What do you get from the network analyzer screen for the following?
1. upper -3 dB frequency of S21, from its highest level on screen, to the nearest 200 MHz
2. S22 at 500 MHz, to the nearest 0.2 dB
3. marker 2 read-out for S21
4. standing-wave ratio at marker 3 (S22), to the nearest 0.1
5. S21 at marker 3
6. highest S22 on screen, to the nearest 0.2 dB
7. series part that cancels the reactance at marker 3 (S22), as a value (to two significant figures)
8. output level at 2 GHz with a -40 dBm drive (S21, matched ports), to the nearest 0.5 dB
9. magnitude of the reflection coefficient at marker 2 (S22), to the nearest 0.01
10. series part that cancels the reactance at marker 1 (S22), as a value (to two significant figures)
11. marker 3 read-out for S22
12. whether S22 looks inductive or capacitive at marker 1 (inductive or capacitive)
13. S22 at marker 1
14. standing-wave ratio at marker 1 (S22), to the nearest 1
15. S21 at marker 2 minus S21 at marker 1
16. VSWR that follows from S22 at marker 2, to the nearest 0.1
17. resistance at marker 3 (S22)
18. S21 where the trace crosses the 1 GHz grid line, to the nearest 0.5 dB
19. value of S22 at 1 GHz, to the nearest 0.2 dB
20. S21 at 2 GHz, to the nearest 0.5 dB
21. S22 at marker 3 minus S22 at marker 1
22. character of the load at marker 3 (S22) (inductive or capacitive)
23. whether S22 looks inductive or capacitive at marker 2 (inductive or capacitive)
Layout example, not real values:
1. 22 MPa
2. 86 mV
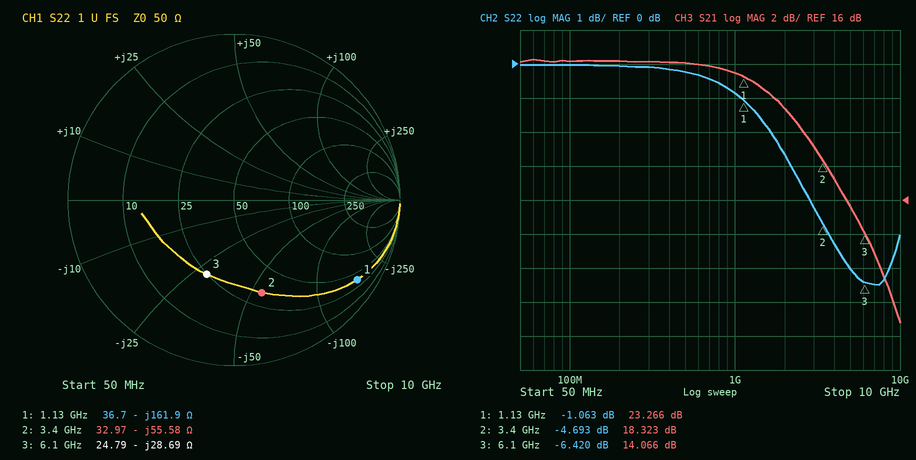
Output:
1. 2.0 GHz
2. -0.2 dB
3. 18.323 dB
4. 2.8
5. 14.066 dB
6. 0.0 dB
7. 750 pH
8. -18.5 dBm
9. 0.58
10. 23 nH
11. -6.420 dB
12. capacitive
13. -1.063 dB
14. 16
15. -4.943 dB
16. 3.8
17. 24.79 Ω
18. 23.5 dB
19. -0.8 dB
20. 21.5 dB
21. -5.357 dB
22. capacitive
23. capacitive
